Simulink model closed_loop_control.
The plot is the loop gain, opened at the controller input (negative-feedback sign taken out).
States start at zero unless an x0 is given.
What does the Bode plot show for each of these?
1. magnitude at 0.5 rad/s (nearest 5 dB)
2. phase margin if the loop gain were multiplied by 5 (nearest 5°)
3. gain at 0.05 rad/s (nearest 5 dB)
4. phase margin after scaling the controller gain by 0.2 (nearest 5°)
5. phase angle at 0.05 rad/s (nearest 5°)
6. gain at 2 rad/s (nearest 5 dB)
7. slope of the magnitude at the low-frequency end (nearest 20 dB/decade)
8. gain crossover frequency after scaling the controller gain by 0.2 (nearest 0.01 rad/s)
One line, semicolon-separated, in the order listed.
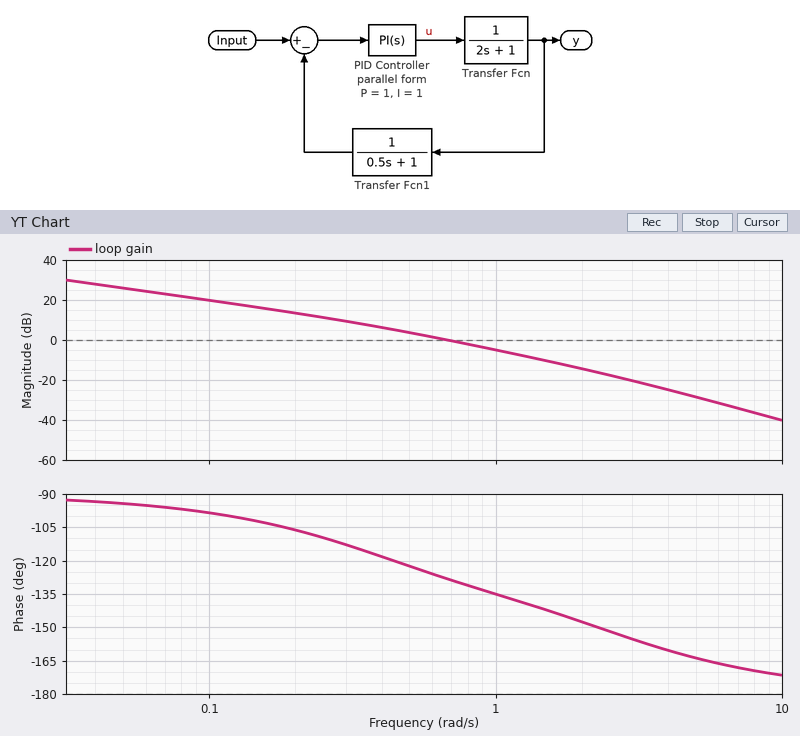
5 dB; 35°; 25 dB; 75°; -95°; -15 dB; -20 dB/decade; 0.19 rad/s
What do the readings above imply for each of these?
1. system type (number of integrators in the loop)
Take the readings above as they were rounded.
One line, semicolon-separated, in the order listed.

1
